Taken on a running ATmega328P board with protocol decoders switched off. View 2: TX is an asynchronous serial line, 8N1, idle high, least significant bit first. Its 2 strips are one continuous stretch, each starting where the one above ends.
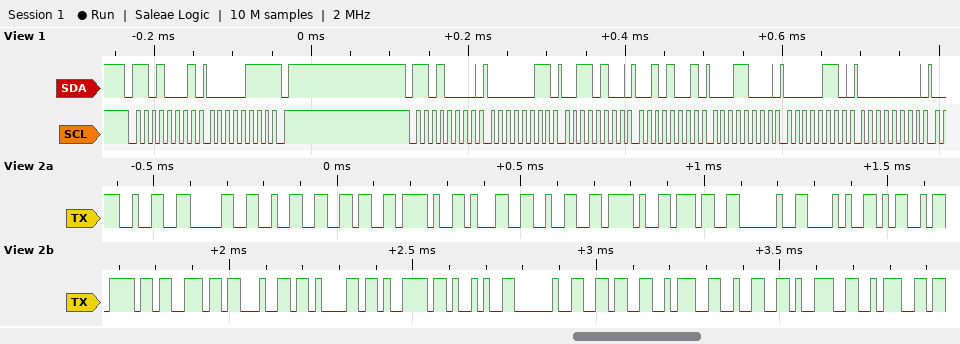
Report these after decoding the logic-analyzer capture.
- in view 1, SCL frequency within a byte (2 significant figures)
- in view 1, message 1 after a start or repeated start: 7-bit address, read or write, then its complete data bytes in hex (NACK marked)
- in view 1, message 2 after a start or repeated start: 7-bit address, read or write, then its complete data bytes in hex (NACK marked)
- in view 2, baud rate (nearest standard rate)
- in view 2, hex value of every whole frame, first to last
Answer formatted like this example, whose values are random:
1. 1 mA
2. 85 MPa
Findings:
1. 100 kHz
2. 0x68 read: 07 NACK
3. 0x68 write: 03 34 29 18 06 00
4. 57600 baud
5. 32 30 32 36 2F 31 32 2F 37 20 28 4D 6F 6E 64 61 79 29 20 36 3A 32 39 3A
